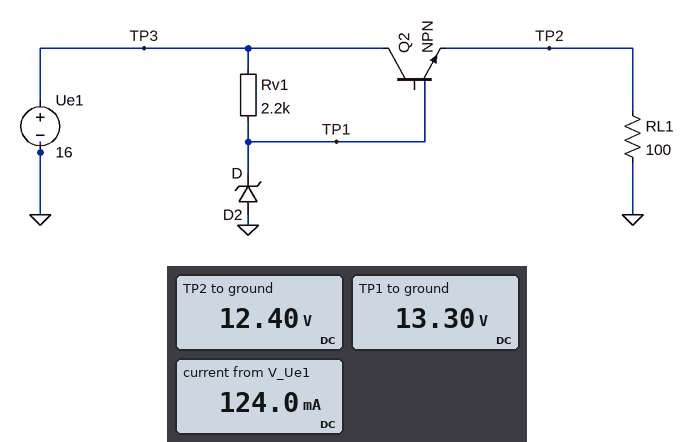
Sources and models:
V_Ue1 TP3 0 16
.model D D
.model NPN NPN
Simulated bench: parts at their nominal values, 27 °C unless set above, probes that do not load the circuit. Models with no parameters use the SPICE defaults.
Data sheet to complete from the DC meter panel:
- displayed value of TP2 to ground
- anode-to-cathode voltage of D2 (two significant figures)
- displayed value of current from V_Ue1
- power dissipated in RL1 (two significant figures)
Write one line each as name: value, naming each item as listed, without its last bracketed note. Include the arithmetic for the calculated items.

displayed value of TP2 to ground: 12.40 V
anode-to-cathode voltage of D2: 0 V - 13.3 V = -13 V
displayed value of current from V_Ue1: 124.0 mA
power dissipated in RL1: (12.4 V)^2 / 100 Ω = 1.5 W
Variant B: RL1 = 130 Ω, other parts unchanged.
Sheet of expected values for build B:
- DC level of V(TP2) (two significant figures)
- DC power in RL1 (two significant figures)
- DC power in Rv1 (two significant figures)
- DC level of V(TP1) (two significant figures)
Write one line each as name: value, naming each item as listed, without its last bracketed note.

DC level of V(TP2): 13 V
DC power in RL1: 1.3 W
DC power in Rv1: 2.1 mW
DC level of V(TP1): 14 V
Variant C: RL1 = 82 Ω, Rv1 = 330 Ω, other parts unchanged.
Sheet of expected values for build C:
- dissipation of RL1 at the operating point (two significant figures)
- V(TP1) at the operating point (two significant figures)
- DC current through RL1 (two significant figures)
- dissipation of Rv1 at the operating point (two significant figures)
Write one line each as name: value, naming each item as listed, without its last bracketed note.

dissipation of RL1 at the operating point: 2.6 W
V(TP1) at the operating point: 15 V
DC current through RL1: 180 mA
dissipation of Rv1 at the operating point: 1.0 mW
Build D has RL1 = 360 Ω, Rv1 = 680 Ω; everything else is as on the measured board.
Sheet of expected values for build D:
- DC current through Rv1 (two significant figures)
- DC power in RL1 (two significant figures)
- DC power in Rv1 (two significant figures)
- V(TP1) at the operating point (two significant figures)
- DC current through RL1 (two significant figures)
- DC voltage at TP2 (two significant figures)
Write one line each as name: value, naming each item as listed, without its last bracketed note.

DC current through Rv1: 410 µA
DC power in RL1: 610 mW
DC power in Rv1: 110 µW
V(TP1) at the operating point: 16 V
DC current through RL1: 41 mA
DC voltage at TP2: 15 V
